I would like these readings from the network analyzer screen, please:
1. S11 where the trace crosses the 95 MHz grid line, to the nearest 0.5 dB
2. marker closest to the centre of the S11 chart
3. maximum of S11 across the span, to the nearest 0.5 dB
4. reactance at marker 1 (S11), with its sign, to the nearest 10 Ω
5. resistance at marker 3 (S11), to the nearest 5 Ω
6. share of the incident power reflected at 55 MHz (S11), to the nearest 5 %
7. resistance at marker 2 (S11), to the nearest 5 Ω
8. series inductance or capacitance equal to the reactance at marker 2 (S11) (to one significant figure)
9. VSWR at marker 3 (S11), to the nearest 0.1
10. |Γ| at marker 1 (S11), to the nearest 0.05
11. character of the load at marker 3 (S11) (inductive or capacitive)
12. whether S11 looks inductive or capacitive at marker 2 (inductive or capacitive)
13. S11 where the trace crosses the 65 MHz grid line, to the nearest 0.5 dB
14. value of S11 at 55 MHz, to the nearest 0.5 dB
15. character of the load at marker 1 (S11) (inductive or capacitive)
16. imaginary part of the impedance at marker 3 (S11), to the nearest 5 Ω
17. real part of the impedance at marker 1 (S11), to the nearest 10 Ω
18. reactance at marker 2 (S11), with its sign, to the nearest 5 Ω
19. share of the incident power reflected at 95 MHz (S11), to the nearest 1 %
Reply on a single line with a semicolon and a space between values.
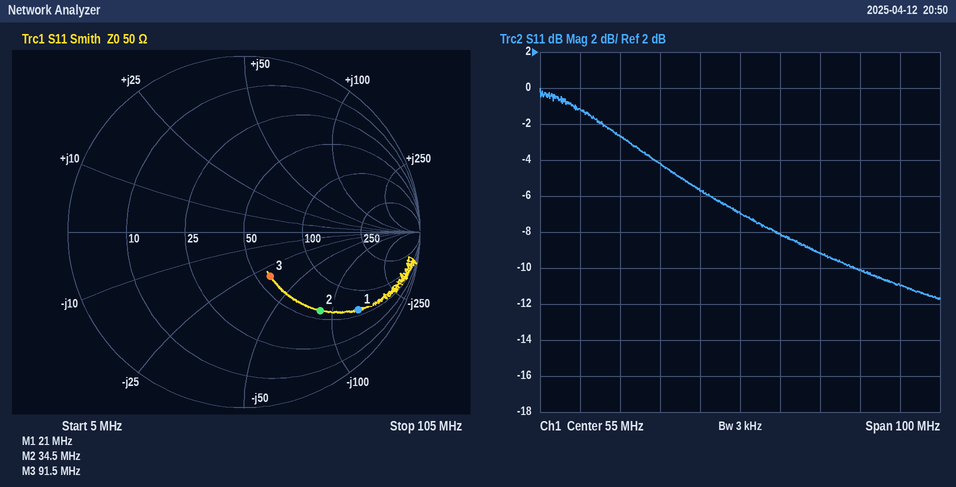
-11.0 dB; marker 3; 0.0 dB; -140 Ω; 60 Ω; 20 %; 60 Ω; 50 pF; 1.8; 0.80; capacitive; capacitive; -8.0 dB; -7.0 dB; capacitive; -30 Ω; 60 Ω; -85 Ω; 8 %
